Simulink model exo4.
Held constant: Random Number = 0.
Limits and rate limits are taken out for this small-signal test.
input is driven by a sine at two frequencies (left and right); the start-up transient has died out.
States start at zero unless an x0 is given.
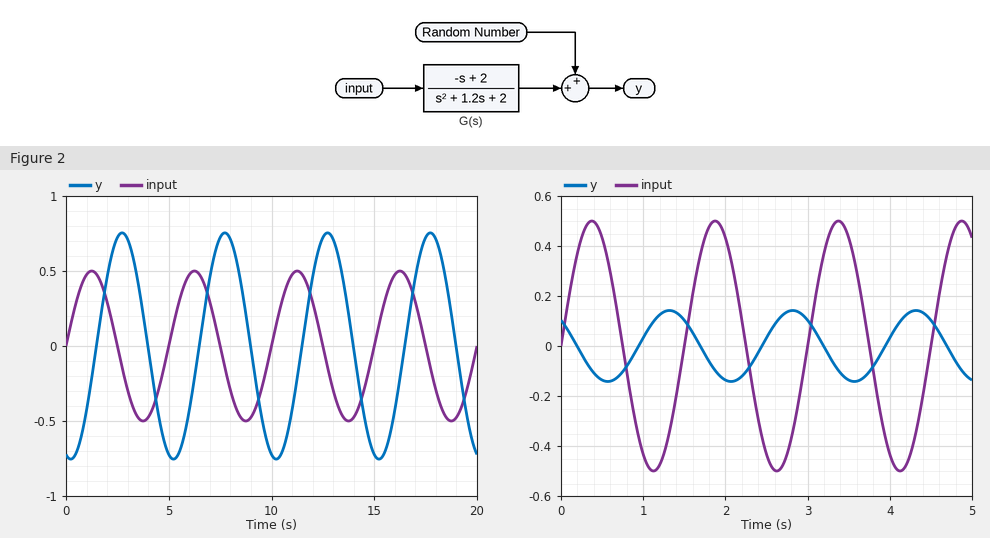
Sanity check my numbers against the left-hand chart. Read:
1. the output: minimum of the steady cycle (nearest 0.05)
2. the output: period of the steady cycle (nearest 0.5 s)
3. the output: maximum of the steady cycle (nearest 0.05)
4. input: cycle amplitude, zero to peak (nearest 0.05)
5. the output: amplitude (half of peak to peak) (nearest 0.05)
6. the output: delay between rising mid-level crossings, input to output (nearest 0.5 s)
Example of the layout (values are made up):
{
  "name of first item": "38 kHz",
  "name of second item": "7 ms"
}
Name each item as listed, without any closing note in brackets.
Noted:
{
  "the output: minimum of the steady cycle": "-0.75",
  "the output: period of the steady cycle": "5.0 s",
  "the output: maximum of the steady cycle": "0.75",
  "input: cycle amplitude, zero to peak": "0.50",
  "the output: amplitude (half of peak to peak)": "0.75",
  "the output: delay between rising mid-level crossings, input to output": "1.5 s"
}
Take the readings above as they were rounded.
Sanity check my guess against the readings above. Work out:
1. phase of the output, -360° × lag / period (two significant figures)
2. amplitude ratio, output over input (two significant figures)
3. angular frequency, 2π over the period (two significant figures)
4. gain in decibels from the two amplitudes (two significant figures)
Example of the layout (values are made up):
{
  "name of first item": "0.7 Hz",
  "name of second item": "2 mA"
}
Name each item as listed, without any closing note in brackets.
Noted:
{
  "phase of the output, -360° × lag / period": "-110°",
  "amplitude ratio, output over input": "1.5",
  "angular frequency, 2π over the period": "1.3 rad/s",
  "gain in decibels from the two amplitudes": "3.5 dB"
}
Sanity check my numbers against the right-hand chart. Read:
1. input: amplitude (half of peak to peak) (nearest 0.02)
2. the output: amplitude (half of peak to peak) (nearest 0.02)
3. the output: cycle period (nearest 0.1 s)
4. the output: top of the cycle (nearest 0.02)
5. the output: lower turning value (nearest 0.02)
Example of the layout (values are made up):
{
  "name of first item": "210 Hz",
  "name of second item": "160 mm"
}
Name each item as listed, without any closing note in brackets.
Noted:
{
  "input: amplitude (half of peak to peak)": "0.50",
  "the output: amplitude (half of peak to peak)": "0.14",
  "the output: cycle period": "1.5 s",
  "the output: top of the cycle": "0.14",
  "the output: lower turning value": "-0.14"
}
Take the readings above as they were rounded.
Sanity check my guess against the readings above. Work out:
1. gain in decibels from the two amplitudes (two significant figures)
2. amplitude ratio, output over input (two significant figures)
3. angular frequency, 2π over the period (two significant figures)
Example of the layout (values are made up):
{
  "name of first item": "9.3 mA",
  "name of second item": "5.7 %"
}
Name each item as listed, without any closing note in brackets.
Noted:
{
  "gain in decibels from the two amplitudes": "-11 dB",
  "amplitude ratio, output over input": "0.28",
  "angular frequency, 2π over the period": "4.2 rad/s"
}
